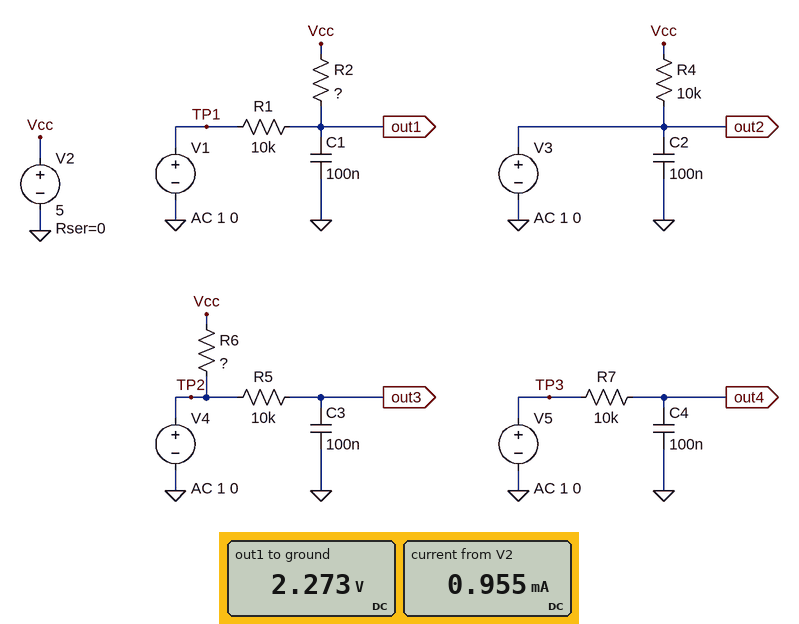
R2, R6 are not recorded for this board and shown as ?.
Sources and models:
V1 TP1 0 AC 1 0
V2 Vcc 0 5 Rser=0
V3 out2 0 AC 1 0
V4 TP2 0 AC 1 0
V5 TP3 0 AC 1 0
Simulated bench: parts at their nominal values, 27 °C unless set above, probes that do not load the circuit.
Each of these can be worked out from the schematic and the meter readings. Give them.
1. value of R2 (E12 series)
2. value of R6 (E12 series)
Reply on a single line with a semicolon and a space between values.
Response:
12 kΩ; 22 kΩ
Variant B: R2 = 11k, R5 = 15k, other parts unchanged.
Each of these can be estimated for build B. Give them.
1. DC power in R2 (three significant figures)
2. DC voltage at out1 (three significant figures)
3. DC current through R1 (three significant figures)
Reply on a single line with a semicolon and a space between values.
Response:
624 µW; 2.38 V; 238 µA
